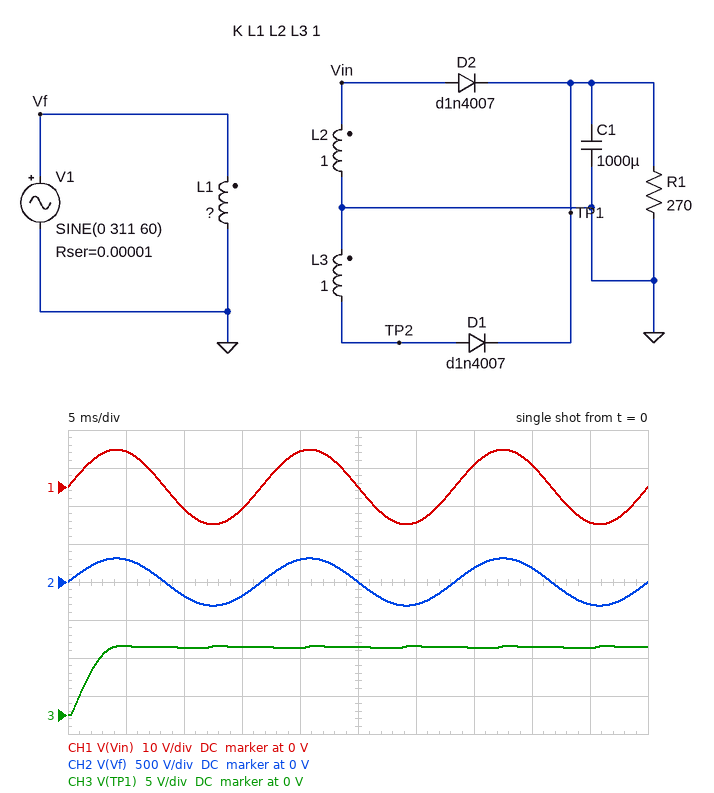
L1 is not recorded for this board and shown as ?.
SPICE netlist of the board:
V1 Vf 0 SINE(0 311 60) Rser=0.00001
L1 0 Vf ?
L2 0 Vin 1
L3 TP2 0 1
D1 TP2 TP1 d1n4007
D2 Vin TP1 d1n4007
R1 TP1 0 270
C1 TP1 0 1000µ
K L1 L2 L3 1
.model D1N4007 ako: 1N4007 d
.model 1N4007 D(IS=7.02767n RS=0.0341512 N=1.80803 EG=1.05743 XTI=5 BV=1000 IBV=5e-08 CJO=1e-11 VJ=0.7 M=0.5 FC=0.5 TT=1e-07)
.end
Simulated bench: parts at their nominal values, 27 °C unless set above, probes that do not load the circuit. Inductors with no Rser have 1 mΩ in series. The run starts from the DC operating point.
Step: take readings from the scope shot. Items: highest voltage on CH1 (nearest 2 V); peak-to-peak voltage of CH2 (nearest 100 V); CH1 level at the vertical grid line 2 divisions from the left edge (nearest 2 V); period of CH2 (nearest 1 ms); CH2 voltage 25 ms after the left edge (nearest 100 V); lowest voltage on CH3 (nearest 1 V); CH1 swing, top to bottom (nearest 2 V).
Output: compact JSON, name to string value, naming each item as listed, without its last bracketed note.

{"highest voltage on CH1": "10 V", "peak-to-peak voltage of CH2": "600 V", "CH1 level at the vertical grid line 2 divisions from the left edge": "-6 V", "period of CH2": "17 ms", "CH2 voltage 25 ms after the left edge": "0 V", "lowest voltage on CH3": "0 V", "CH1 swing, top to bottom": "20 V"}
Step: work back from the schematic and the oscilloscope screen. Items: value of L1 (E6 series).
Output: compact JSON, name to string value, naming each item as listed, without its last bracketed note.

{"value of L1": "1 kH"}
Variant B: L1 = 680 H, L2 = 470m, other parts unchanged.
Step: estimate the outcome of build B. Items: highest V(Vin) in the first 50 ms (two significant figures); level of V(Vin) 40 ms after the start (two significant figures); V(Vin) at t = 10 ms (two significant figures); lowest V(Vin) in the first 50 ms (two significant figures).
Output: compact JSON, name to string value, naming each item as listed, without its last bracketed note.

{"highest V(Vin) in the first 50 ms": "8.2 V", "level of V(Vin) 40 ms after the start": "4.8 V", "V(Vin) at t = 10 ms": "-4.8 V", "lowest V(Vin) in the first 50 ms": "-8.2 V"}
